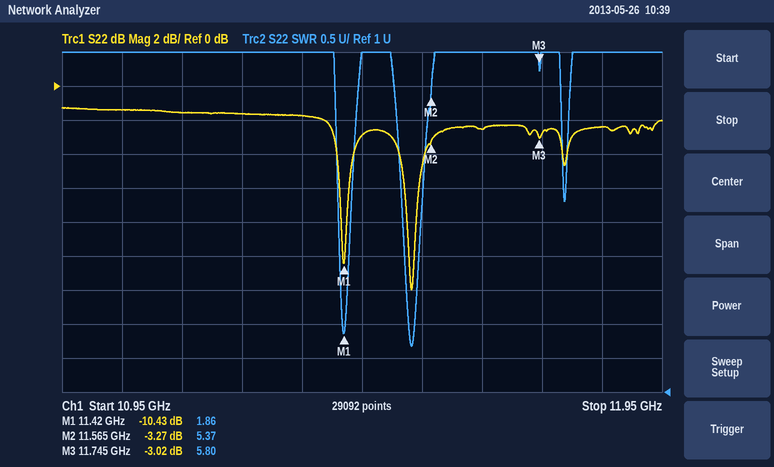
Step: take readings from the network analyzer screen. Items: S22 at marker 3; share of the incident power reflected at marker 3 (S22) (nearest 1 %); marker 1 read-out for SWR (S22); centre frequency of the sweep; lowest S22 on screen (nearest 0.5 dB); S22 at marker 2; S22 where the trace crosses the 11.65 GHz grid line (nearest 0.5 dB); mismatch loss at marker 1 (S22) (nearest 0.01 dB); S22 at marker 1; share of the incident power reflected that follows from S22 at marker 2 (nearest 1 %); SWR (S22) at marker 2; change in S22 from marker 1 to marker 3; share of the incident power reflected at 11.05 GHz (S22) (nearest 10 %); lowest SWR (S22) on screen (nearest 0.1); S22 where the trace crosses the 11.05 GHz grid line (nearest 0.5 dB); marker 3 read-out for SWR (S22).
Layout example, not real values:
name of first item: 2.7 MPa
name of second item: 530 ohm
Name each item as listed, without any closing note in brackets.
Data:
S22 at marker 3: -3.02 dB
share of the incident power reflected at marker 3 (S22): 50 %
marker 1 read-out for SWR: 1.86
centre frequency of the sweep: 11.45 GHz
lowest S22 on screen: -12.0 dB
S22 at marker 2: -3.27 dB
S22 where the trace crosses the 11.65 GHz grid line: -2.5 dB
mismatch loss at marker 1 (S22): 0.41 dB
S22 at marker 1: -10.43 dB
share of the incident power reflected that follows from S22 at marker 2: 47 %
SWR (S22) at marker 2: 5.37
change in S22 from marker 1 to marker 3: 7.41 dB
share of the incident power reflected at 11.05 GHz (S22): 70 %
lowest SWR (S22) on screen: 1.7
S22 where the trace crosses the 11.05 GHz grid line: -1.5 dB
marker 3 read-out for SWR: 5.80
